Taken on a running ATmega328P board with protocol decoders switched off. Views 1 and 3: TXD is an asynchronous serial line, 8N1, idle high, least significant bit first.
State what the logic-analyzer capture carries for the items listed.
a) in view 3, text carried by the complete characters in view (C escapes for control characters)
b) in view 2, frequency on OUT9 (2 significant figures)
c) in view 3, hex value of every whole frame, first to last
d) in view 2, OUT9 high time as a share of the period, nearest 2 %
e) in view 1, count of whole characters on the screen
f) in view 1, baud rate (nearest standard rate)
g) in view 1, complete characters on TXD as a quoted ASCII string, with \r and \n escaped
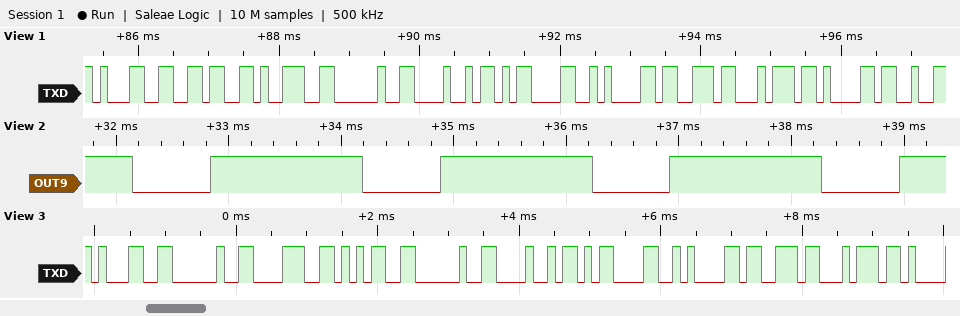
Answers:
"1 85 H\r\nst"
490 Hz
31 20 38 35 20 48 0D 0A 73 74
66 %
10
9600 baud
"169 H\r\nsta"
